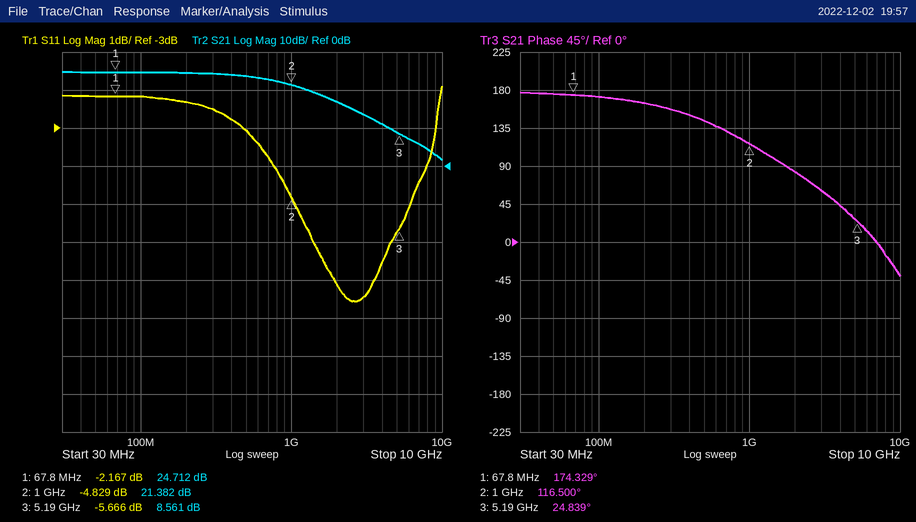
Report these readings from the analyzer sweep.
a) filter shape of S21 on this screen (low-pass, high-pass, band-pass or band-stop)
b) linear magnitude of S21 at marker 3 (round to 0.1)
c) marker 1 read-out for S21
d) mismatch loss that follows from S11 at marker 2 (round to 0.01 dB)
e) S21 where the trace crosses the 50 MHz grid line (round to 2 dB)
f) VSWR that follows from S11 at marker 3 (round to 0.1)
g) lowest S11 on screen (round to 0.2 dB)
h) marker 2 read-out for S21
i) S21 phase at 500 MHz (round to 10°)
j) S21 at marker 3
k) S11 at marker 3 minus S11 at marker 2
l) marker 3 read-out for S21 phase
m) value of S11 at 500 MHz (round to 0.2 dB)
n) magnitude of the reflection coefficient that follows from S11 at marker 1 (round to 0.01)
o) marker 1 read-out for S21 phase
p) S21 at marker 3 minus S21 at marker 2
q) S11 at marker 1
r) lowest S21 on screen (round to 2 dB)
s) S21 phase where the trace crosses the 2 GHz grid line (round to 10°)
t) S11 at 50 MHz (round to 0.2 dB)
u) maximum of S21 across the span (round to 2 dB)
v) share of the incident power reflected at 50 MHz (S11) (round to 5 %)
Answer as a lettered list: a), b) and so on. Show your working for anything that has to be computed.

a) low-pass
b) 10^(8.561/20) ≈ 2.7
c) 24.712 dB
d) −10 log10(1 − 10^(-4.829/10)) ≈ 1.73 dB
e) 24 dB
f) (1 + 0.5208)/(1 − 0.5208) ≈ 3.2
g) -7.6 dB
h) 21.382 dB
i) 140°
j) 8.561 dB
k) -5.666 − (-4.829) = -0.837 dB
l) 24.839°
m) -3.0 dB
n) 10^(-2.167/20) ≈ 0.78
o) 174.329°
p) 8.561 − (21.382) = -12.821 dB
q) -2.167 dB
r) 2 dB
s) 80°
t) -2.2 dB
u) 24 dB
v) 10^(-2.2/10) ≈ 60 %
